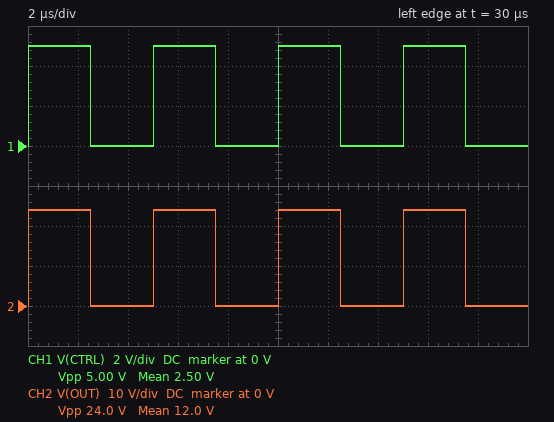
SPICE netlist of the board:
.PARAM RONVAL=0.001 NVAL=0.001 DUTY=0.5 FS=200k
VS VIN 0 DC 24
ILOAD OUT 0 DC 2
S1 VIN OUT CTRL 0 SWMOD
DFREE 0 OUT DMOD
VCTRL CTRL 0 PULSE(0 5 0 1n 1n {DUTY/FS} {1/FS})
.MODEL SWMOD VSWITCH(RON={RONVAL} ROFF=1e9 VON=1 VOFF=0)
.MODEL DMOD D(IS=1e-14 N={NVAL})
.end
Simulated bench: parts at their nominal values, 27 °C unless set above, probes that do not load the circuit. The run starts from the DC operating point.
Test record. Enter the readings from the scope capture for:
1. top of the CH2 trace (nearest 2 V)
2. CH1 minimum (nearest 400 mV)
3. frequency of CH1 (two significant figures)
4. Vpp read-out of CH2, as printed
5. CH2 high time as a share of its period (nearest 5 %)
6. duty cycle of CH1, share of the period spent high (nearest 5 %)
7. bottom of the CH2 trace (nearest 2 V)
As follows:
24 V
0 V
200 kHz
24.0 V
50 %
50 %
0 V
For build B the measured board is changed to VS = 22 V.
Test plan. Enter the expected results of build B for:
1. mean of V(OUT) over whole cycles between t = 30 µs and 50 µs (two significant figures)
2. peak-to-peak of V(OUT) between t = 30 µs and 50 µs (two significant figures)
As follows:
11 V
22 V
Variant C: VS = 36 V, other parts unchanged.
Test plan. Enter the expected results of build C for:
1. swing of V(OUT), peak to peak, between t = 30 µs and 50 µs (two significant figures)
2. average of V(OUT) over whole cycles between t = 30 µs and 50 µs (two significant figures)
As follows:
36 V
18 V
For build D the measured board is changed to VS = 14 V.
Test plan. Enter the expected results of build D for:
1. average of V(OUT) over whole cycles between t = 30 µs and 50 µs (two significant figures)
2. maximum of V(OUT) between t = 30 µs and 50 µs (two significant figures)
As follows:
7.0 V
14 V
